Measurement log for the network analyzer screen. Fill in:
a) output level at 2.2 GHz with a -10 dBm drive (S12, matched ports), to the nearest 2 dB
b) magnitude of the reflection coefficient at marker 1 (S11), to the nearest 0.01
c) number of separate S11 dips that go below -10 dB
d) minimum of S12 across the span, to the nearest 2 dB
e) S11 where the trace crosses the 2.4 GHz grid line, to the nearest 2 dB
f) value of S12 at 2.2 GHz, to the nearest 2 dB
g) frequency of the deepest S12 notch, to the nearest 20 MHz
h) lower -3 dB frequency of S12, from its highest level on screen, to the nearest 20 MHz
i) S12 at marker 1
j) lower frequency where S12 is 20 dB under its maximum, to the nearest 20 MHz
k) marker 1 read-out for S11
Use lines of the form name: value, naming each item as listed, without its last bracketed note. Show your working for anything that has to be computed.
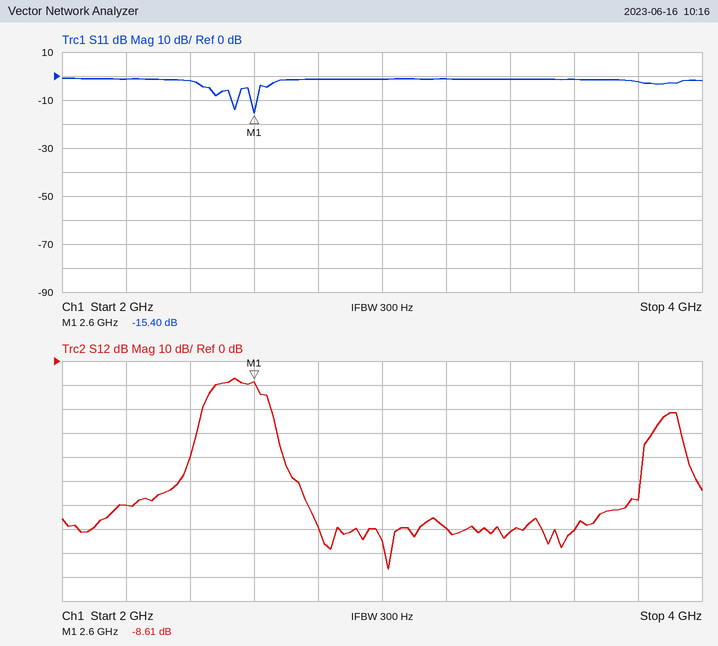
output level at 2.2 GHz with a -10 dBm drive (S12, matched ports), to the nearest 2 dB: -10 dBm + (-60 dB) = -70 dBm
magnitude of the reflection coefficient at marker 1 (S11), to the nearest 0.01: 10^(-15.4/20) ≈ 0.17
number of separate S11 dips that go below -10 dB: 2
minimum of S12 across the span, to the nearest 2 dB: -86 dB
S11 where the trace crosses the 2.4 GHz grid line, to the nearest 2 dB: -2 dB
value of S12 at 2.2 GHz, to the nearest 2 dB: -60 dB
frequency of the deepest S12 notch, to the nearest 20 MHz: 3.02 GHz
lower -3 dB frequency of S12, from its highest level on screen, to the nearest 20 MHz: 2.48 GHz
S12 at marker 1: -8.61 dB
lower frequency where S12 is 20 dB under its maximum, to the nearest 20 MHz: 2.42 GHz
marker 1 read-out for S11: -15.40 dB
